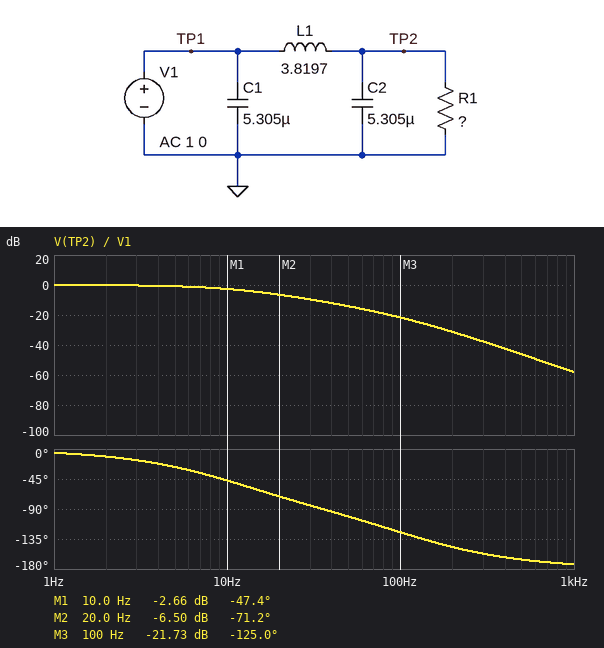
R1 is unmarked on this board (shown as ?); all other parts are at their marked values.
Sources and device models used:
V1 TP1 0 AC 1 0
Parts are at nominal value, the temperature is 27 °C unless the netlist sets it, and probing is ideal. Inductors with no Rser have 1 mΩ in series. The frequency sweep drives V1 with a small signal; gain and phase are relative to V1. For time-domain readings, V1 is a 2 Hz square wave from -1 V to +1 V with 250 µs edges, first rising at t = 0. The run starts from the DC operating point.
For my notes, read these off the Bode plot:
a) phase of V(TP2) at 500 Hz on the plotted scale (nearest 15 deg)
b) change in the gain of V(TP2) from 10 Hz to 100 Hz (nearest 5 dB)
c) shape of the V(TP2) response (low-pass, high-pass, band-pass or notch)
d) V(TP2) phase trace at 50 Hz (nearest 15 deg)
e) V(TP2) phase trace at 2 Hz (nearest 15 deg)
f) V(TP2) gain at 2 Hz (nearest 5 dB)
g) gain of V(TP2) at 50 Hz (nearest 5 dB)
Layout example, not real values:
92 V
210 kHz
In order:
-165 deg
-20 dB
low-pass
-105 deg
-15 deg
0 dB
-15 dB
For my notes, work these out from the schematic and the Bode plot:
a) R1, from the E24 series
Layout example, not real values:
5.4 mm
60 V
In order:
240 Ω
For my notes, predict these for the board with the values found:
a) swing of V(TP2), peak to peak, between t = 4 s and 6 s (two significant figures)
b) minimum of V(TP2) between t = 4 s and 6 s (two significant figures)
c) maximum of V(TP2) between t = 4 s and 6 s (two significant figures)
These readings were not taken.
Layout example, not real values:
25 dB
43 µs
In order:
2.0 V
-1.0 V
1.0 V
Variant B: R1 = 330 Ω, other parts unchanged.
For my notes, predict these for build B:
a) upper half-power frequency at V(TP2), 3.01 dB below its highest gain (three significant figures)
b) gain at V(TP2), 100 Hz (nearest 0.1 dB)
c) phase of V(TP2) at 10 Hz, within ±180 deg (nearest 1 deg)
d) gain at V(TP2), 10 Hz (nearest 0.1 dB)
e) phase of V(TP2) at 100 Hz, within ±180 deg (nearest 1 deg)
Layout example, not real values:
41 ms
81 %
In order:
16.1 Hz
-20.1 dB
-38 deg
-1.4 dB
-134 deg
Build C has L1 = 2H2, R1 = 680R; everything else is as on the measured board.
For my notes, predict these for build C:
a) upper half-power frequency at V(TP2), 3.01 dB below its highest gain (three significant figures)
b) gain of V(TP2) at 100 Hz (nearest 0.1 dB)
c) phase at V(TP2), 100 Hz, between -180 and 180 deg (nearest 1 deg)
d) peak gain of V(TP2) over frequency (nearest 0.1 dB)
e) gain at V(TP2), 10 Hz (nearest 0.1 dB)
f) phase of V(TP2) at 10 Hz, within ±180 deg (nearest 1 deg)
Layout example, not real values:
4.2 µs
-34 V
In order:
54.8 Hz
-12.3 dB
-151 deg
1.6 dB
0.2 dB
-12 deg
